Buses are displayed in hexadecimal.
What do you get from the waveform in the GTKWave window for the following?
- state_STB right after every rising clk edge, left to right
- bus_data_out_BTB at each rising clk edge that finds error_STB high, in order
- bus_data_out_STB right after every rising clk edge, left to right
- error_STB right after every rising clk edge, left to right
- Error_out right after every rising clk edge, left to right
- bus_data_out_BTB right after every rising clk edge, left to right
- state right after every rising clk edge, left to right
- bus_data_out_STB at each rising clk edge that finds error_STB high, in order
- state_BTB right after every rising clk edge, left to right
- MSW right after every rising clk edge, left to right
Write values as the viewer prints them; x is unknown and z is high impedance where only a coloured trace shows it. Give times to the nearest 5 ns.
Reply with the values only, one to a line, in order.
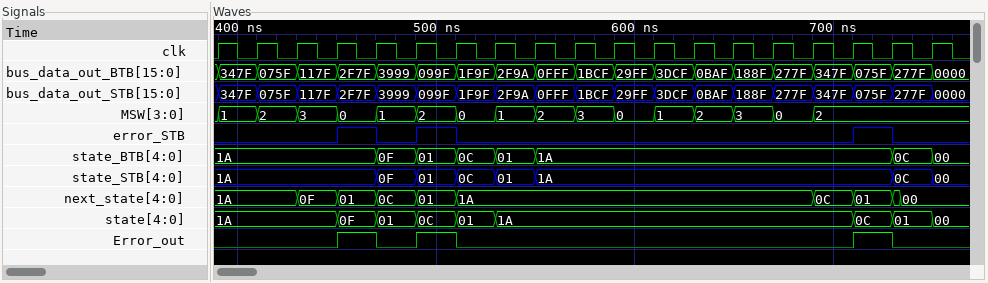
1A, 1A, 1A, 1A, 0F, 01, 0C, 01, 1A, 1A, 1A, 1A, 1A, 1A, 1A, 1A, 1A, 0C, 00
2F7F, 099F, 075F
347F, 075F, 117F, 2F7F, 3999, 099F, 1F9F, 2F9A, 0FFF, 1BCF, 29FF, 3DCF, 0BAF, 188F, 277F, 347F, 075F, 277F, 0000
0 0 0 1 0 1 0 0 0 0 0 0 0 0 0 0 1 0 0
0 0 0 1 0 1 0 0 0 0 0 0 0 0 0 0 1 0 0
347F, 075F, 117F, 2F7F, 3999, 099F, 1F9F, 2F9A, 0FFF, 1BCF, 29FF, 3DCF, 0BAF, 188F, 277F, 347F, 075F, 277F, 0000
1A, 1A, 1A, 0F, 01, 0C, 01, 1A, 1A, 1A, 1A, 1A, 1A, 1A, 1A, 1A, 0C, 01, 00
2F7F, 099F, 075F
1A, 1A, 1A, 1A, 0F, 01, 0C, 01, 1A, 1A, 1A, 1A, 1A, 1A, 1A, 1A, 1A, 0C, 00
1, 2, 3, 0, 1, 2, 0, 1, 2, 3, 0, 1, 2, 3, 0, 2, 2, 2, 2
